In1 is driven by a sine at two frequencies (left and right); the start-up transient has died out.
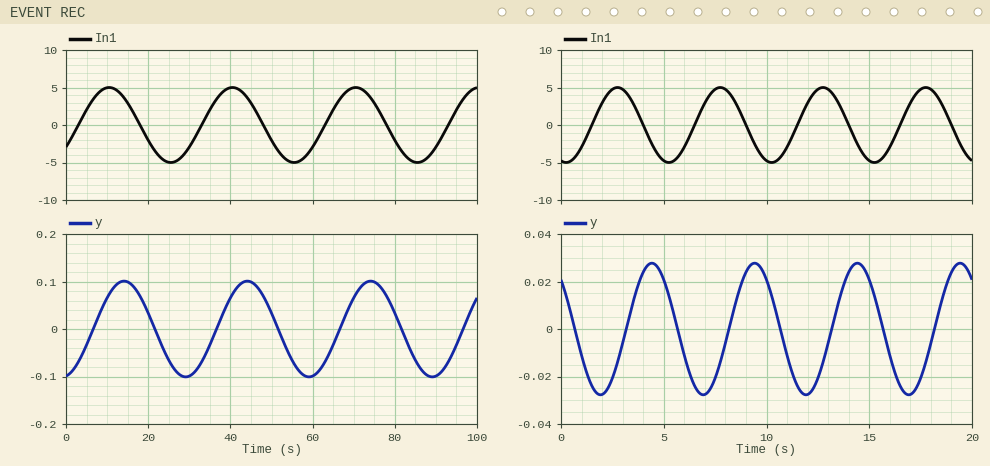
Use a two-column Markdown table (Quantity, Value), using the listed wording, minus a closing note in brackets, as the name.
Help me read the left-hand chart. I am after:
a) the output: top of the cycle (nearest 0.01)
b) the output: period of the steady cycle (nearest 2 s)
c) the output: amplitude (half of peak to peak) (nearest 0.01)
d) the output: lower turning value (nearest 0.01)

| Quantity | Value |
|---|---|
| the output: top of the cycle | 0.10 |
| the output: period of the steady cycle | 30 s |
| the output: amplitude (half of peak to peak) | 0.10 |
| the output: lower turning value | -0.10 |
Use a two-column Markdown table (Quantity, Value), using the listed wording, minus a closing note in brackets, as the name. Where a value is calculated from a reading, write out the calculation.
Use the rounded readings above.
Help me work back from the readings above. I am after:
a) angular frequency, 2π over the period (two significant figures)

| Quantity | Value |
|---|---|
| angular frequency, 2π over the period | 2π / 30 = 0.21 rad/s |
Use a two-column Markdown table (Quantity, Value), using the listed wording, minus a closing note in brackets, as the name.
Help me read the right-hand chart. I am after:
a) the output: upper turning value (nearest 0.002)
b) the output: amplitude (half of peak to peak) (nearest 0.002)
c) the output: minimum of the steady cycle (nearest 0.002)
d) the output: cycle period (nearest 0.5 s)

| Quantity | Value |
|---|---|
| the output: upper turning value | 0.028 |
| the output: amplitude (half of peak to peak) | 0.028 |
| the output: minimum of the steady cycle | -0.028 |
| the output: cycle period | 5.0 s |
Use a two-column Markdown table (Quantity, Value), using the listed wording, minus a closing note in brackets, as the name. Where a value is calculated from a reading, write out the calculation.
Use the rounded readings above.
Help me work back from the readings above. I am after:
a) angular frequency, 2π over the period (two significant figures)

| Quantity | Value |
|---|---|
| angular frequency, 2π over the period | 2π / 5 = 1.3 rad/s |
